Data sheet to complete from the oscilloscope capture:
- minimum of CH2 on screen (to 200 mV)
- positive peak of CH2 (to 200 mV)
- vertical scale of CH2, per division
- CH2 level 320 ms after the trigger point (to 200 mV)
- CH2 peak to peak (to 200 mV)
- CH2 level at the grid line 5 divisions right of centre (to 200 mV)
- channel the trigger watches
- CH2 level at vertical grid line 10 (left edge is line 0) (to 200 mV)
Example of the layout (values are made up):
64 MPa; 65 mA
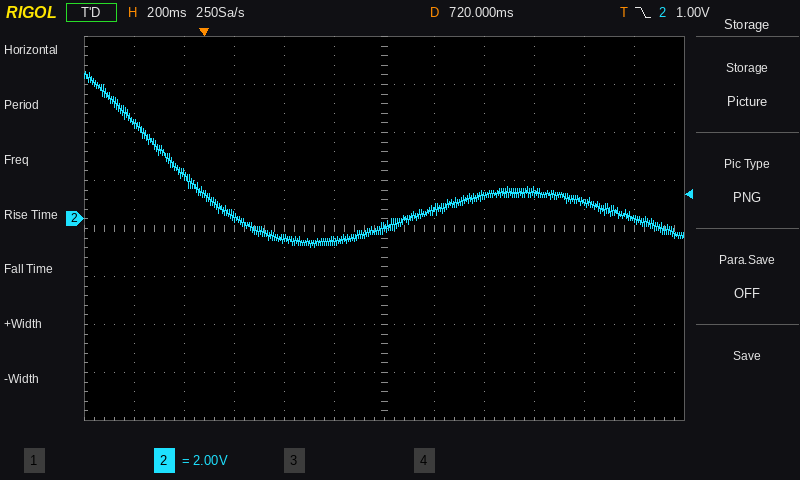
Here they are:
-1.2 V; 6.2 V; 2 V; -800 mV; 7.4 V; 0.0 V; CH2; 600 mV
